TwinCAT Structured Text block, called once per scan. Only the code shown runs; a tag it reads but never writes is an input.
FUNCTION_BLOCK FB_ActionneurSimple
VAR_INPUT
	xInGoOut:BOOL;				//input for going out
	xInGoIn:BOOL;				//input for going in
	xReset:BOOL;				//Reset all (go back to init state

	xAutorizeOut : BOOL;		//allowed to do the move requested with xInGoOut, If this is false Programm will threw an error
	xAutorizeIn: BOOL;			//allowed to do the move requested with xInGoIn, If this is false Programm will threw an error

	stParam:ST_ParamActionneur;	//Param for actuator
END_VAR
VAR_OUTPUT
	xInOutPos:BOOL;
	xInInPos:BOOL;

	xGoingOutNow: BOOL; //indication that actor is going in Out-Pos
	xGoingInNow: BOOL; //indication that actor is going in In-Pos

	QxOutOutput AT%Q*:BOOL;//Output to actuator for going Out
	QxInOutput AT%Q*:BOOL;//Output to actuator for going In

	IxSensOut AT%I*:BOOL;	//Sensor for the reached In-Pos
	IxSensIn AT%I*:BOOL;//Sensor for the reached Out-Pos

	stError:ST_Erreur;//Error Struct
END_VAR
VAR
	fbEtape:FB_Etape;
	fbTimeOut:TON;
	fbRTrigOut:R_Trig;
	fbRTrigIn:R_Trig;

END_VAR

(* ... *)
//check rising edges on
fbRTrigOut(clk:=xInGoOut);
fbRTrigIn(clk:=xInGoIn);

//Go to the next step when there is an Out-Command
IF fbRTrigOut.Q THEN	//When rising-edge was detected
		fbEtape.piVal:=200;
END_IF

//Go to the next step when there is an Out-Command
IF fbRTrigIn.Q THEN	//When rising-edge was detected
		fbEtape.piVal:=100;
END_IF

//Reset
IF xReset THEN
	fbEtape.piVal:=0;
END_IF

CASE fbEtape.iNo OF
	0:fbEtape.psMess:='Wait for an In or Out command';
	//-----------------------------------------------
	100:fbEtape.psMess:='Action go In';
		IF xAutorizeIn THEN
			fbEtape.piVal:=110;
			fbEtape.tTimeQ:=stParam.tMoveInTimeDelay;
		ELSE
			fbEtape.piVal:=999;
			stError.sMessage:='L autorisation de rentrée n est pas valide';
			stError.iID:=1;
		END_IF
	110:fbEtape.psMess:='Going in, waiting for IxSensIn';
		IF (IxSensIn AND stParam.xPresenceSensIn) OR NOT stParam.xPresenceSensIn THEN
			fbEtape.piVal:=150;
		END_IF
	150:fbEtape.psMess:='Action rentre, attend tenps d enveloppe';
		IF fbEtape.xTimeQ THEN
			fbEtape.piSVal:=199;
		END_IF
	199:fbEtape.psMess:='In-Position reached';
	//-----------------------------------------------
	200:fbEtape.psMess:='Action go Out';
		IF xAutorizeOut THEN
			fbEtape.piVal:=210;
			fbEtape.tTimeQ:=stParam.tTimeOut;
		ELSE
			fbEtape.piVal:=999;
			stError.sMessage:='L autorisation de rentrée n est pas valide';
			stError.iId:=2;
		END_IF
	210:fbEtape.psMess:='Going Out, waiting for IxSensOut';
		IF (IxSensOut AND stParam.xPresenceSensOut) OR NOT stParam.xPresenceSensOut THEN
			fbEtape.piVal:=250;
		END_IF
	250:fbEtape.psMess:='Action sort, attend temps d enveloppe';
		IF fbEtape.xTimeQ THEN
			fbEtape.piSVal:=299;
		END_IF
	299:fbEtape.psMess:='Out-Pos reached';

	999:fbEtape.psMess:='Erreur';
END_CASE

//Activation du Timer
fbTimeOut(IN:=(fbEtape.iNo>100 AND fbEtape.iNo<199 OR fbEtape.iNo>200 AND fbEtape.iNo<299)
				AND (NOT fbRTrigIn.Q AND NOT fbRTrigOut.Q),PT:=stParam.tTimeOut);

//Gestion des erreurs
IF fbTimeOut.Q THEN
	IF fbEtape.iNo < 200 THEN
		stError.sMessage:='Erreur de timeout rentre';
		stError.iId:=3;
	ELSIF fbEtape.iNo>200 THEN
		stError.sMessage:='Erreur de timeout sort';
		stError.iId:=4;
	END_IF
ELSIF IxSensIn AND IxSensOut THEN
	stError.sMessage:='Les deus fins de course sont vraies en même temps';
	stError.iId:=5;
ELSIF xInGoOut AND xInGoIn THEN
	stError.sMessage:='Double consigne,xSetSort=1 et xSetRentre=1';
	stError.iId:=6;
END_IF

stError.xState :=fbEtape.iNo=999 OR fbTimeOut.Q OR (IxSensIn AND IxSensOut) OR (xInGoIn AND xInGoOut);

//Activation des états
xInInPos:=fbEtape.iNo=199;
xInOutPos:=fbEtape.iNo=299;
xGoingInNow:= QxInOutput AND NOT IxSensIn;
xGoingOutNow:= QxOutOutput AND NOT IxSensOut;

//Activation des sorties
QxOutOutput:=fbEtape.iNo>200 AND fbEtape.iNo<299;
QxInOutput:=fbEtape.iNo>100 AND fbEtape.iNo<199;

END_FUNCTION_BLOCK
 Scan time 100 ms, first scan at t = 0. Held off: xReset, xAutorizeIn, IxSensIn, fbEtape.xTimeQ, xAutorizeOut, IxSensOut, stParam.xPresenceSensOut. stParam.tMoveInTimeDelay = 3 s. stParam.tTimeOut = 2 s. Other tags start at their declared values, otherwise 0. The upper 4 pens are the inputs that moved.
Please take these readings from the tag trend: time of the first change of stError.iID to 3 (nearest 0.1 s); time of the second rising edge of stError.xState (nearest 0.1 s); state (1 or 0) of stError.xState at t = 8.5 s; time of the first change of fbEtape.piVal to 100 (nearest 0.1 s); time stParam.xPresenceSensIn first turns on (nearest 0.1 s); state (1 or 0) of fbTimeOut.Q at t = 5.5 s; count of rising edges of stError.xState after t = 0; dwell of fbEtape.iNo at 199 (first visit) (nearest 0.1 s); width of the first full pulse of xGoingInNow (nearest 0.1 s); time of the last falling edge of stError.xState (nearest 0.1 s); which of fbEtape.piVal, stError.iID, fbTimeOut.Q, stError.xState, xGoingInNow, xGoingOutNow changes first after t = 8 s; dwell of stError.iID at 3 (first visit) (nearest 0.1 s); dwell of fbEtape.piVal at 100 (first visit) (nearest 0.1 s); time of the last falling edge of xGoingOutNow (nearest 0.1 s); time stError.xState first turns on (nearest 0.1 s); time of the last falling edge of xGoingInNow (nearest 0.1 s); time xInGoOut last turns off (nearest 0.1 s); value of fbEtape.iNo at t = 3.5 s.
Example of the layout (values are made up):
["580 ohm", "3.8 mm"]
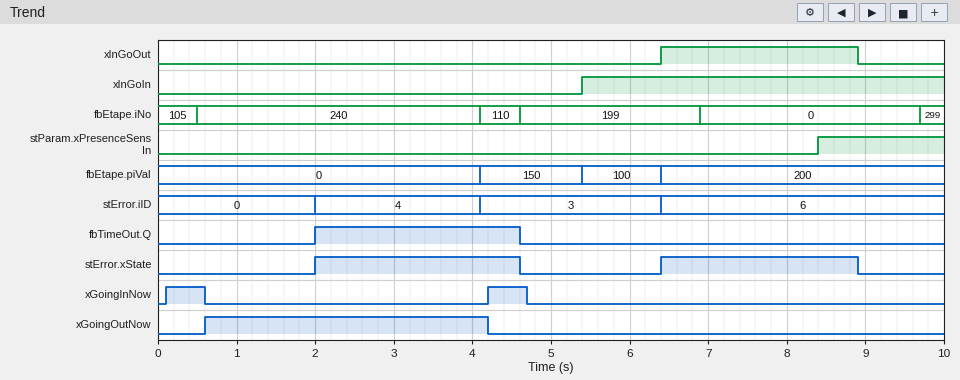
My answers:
["4.1 s", "6.4 s", "1", "5.4 s", "8.4 s", "0", "2", "2.3 s", "0.5 s", "8.9 s", "stError.xState", "2.3 s", "1.0 s", "4.2 s", "2.0 s", "4.7 s", "8.9 s", "240"]
